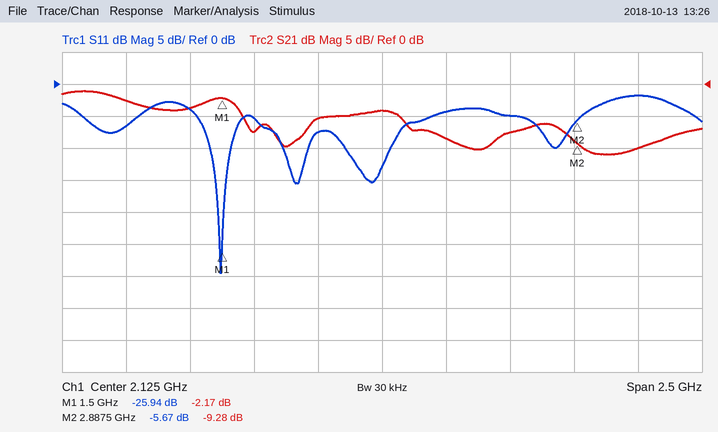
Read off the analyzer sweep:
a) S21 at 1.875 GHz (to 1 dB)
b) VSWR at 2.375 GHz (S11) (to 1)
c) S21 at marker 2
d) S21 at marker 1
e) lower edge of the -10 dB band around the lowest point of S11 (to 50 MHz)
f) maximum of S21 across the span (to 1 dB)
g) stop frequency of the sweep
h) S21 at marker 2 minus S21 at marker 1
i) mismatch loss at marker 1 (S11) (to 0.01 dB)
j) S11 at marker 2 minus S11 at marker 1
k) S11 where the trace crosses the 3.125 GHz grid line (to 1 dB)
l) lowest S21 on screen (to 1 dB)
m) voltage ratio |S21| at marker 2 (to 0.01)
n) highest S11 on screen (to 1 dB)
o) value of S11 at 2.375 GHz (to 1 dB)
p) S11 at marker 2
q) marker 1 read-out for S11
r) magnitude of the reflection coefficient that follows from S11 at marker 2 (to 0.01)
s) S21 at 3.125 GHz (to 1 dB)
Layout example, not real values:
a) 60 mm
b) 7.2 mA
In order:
a) -5 dB
b) 4
c) -9.28 dB
d) -2.17 dB
e) 1.45 GHz
f) -1 dB
g) 3.375 GHz
h) -7.11 dB
i) 0.01 dB
j) 20.27 dB
k) -2 dB
l) -11 dB
m) 0.34
n) -2 dB
o) -4 dB
p) -5.67 dB
q) -25.94 dB
r) 0.52
s) -10 dB
